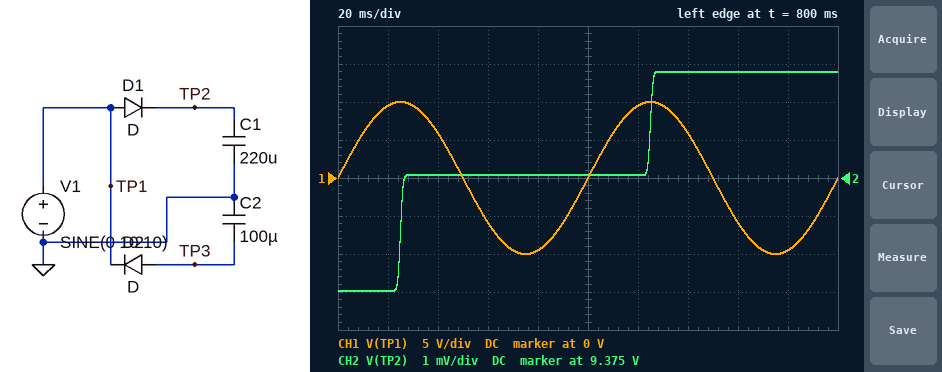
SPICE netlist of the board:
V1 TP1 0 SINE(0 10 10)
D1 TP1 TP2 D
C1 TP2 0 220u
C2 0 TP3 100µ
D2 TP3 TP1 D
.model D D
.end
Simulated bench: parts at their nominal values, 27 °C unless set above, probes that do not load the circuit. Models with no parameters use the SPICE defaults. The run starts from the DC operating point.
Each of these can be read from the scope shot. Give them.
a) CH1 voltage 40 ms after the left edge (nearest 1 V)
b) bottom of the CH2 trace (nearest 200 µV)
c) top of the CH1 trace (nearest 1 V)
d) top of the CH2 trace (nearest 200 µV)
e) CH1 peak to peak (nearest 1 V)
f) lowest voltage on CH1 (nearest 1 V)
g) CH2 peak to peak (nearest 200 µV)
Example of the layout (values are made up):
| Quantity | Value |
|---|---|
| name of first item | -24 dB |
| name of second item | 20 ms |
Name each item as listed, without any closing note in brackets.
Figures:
| Quantity | Value |
|---|---|
| CH1 voltage 40 ms after the left edge | 6 V |
| bottom of the CH2 trace | 9.3720 V |
| top of the CH1 trace | 10 V |
| top of the CH2 trace | 9.3778 V |
| CH1 peak to peak | 20 V |
| lowest voltage on CH1 | -10 V |
| CH2 peak to peak | 5.8 mV |
